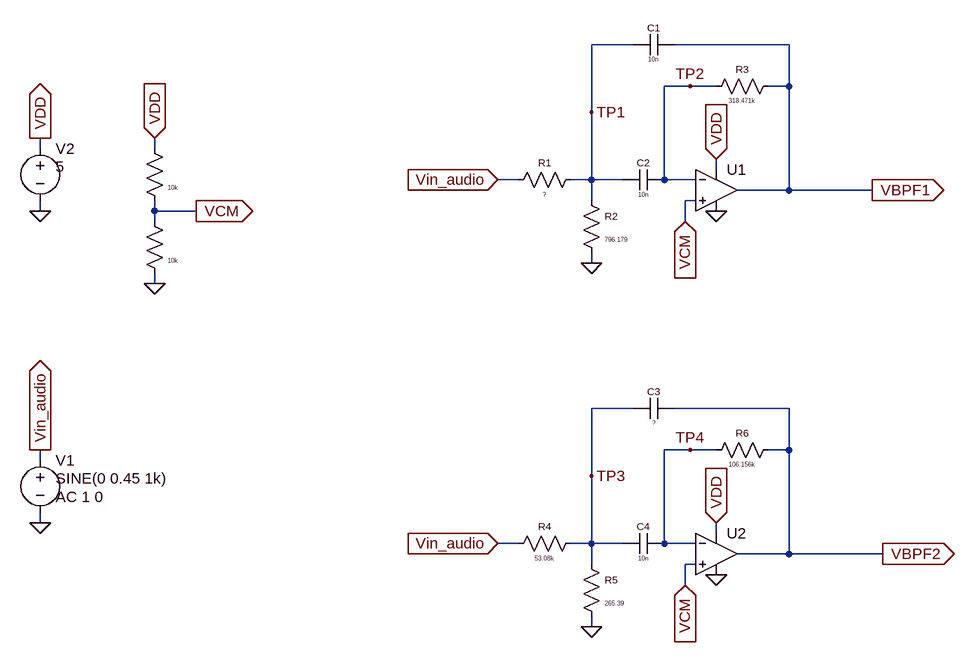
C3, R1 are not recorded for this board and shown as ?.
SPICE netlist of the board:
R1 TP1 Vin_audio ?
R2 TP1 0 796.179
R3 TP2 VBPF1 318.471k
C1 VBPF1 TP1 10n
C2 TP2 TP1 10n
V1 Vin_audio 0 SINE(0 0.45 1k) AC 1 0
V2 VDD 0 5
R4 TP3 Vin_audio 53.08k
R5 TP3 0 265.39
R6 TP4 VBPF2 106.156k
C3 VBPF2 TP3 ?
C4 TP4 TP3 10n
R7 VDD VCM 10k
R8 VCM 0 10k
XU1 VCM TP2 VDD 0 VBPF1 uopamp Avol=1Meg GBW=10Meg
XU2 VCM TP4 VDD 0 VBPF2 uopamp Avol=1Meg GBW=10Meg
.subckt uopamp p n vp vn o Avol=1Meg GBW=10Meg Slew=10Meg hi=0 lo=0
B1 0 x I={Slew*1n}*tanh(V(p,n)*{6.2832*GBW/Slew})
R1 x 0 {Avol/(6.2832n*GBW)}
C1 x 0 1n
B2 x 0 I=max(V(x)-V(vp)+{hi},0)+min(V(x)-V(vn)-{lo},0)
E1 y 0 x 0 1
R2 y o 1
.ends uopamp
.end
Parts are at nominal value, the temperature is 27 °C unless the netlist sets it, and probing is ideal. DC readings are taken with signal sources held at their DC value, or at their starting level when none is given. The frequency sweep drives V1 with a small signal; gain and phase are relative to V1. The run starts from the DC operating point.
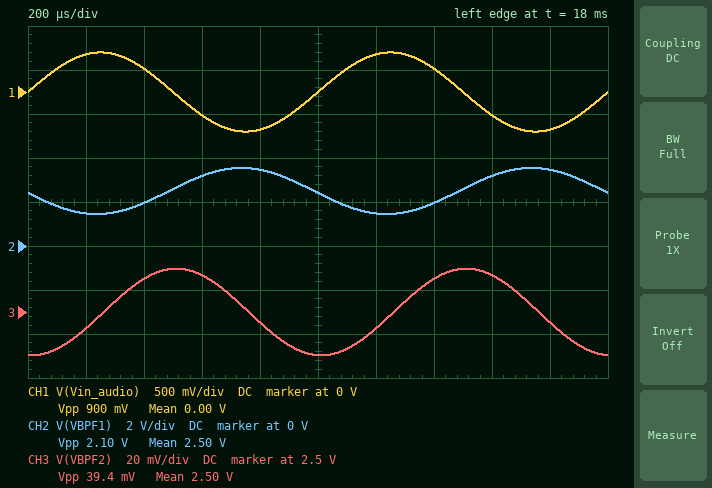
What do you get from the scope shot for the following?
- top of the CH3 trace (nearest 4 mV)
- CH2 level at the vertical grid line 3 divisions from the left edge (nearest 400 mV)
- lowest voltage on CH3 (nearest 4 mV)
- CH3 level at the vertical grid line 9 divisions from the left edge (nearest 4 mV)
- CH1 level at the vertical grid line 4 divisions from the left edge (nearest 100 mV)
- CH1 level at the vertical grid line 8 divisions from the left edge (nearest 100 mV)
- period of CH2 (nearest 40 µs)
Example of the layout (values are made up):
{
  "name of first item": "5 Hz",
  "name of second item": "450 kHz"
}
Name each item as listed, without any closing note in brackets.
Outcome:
{
  "top of the CH3 trace": "2.520 V",
  "CH2 level at the vertical grid line 3 divisions from the left edge": "3.2 V",
  "lowest voltage on CH3": "2.480 V",
  "CH3 level at the vertical grid line 9 divisions from the left edge": "2.496 V",
  "CH1 level at the vertical grid line 4 divisions from the left edge": "-400 mV",
  "CH1 level at the vertical grid line 8 divisions from the left edge": "-300 mV",
  "period of CH2": "1.00 ms"
}
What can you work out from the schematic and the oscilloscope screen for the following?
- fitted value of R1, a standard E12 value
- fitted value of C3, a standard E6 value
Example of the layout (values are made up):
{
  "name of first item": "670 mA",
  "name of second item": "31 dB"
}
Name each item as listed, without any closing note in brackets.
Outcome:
{
  "fitted value of R1, a standard E12 value": "68 kΩ",
  "fitted value of C3, a standard E6 value": "22 nF"
}
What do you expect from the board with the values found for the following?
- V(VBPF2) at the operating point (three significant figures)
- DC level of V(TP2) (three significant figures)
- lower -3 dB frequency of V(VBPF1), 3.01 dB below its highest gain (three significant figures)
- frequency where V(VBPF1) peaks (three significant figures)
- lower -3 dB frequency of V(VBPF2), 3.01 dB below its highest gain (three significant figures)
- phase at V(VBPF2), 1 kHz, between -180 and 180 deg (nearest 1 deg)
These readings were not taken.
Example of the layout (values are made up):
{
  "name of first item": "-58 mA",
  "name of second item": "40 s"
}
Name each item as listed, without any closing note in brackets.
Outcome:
{
  "V(VBPF2) at the operating point": "2.50 V",
  "DC level of V(TP2)": "2.50 V",
  "lower -3 dB frequency of V(VBPF1), 3.01 dB below its highest gain": "956 Hz",
  "frequency where V(VBPF1) peaks": "1.00 kHz",
  "lower -3 dB frequency of V(VBPF2), 3.01 dB below its highest gain": "1.92 kHz",
  "phase at V(VBPF2), 1 kHz, between -180 and 180 deg": "-94 deg"
}
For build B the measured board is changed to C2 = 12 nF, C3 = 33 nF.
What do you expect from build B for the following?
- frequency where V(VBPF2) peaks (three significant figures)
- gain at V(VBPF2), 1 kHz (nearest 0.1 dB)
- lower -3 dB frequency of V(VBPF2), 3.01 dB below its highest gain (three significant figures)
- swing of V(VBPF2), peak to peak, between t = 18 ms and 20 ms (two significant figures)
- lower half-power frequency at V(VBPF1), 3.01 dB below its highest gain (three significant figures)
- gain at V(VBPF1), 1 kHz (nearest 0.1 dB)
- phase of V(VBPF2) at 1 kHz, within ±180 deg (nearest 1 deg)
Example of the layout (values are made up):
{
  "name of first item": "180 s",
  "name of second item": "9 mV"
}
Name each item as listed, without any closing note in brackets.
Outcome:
{
  "frequency where V(VBPF2) peaks": "1.65 kHz",
  "gain at V(VBPF2), 1 kHz": "-25.7 dB",
  "lower -3 dB frequency of V(VBPF2), 3.01 dB below its highest gain": "1.56 kHz",
  "swing of V(VBPF2), peak to peak, between t = 18 ms and 20 ms": "47 mV",
  "lower half-power frequency at V(VBPF1), 3.01 dB below its highest gain": "872 Hz",
  "gain at V(VBPF1), 1 kHz": "2.1 dB",
  "phase of V(VBPF2) at 1 kHz, within ±180 deg": "-96 deg"
}
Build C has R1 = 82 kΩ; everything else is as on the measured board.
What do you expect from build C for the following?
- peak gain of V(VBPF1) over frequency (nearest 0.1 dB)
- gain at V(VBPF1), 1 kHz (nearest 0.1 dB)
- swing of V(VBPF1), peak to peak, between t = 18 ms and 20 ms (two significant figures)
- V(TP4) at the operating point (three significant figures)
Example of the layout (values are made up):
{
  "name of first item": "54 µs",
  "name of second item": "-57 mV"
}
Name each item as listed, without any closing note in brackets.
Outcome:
{
  "peak gain of V(VBPF1) over frequency": "5.8 dB",
  "gain at V(VBPF1), 1 kHz": "5.7 dB",
  "swing of V(VBPF1), peak to peak, between t = 18 ms and 20 ms": "1.7 V",
  "V(TP4) at the operating point": "2.50 V"
}
